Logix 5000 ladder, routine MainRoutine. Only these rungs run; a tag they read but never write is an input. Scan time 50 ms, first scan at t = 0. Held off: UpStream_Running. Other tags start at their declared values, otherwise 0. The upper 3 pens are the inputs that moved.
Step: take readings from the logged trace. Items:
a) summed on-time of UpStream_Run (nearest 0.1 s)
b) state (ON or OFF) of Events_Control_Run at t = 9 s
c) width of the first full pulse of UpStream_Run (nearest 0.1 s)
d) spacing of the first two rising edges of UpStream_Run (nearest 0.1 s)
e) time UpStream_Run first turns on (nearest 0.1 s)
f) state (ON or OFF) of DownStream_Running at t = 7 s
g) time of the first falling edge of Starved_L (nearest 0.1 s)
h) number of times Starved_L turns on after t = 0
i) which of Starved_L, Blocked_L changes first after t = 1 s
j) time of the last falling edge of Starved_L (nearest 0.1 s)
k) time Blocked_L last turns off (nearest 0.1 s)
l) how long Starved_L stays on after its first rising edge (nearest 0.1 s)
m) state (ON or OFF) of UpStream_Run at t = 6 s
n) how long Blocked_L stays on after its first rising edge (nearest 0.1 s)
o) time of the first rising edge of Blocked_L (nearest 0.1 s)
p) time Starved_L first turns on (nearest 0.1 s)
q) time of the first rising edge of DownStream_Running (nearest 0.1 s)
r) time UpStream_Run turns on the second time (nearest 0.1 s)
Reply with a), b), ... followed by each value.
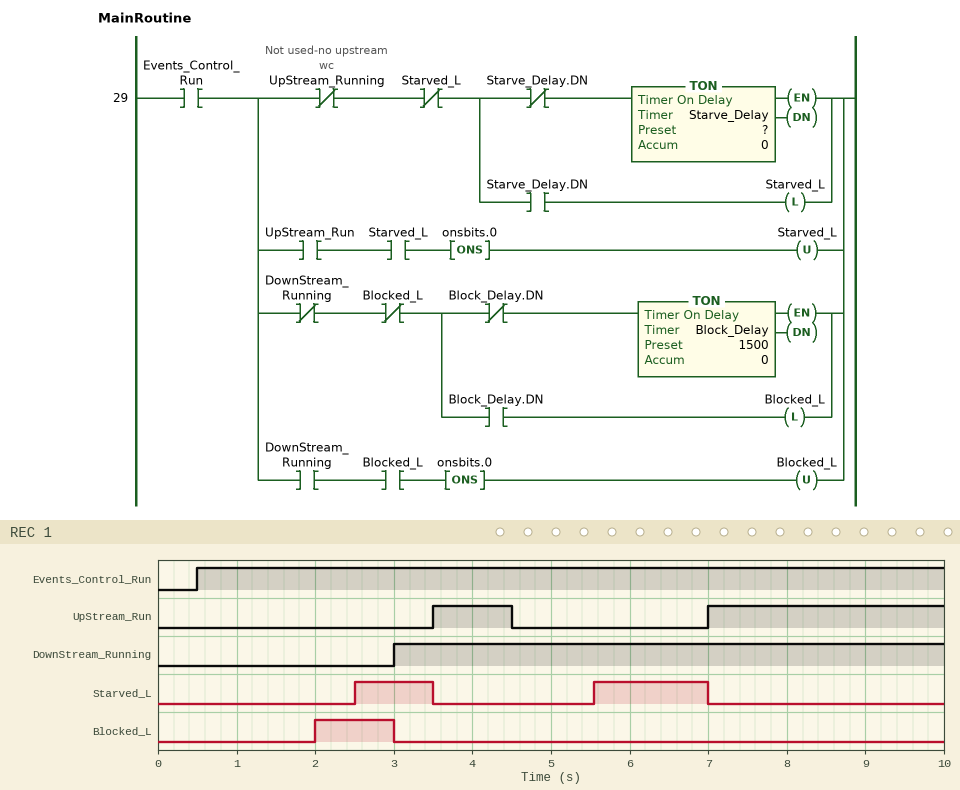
a) 4.0 s
b) ON
c) 1.0 s
d) 3.5 s
e) 3.5 s
f) ON
g) 3.5 s
h) 2
i) Blocked_L
j) 7.0 s
k) 3.0 s
l) 1.0 s
m) OFF
n) 1.0 s
o) 2.0 s
p) 2.5 s
q) 3.0 s
r) 7.0 s
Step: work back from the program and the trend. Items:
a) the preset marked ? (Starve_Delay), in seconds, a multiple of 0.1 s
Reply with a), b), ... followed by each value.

a) 2.0 s
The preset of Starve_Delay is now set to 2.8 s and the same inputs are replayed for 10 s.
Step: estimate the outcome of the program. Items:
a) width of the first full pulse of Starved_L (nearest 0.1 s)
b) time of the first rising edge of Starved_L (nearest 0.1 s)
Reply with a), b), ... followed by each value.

a) 0.2 s
b) 3.3 s
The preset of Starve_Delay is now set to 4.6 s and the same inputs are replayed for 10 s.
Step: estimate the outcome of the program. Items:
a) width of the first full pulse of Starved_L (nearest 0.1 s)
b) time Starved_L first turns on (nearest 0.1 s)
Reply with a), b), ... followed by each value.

a) 1.9 s
b) 5.1 s
